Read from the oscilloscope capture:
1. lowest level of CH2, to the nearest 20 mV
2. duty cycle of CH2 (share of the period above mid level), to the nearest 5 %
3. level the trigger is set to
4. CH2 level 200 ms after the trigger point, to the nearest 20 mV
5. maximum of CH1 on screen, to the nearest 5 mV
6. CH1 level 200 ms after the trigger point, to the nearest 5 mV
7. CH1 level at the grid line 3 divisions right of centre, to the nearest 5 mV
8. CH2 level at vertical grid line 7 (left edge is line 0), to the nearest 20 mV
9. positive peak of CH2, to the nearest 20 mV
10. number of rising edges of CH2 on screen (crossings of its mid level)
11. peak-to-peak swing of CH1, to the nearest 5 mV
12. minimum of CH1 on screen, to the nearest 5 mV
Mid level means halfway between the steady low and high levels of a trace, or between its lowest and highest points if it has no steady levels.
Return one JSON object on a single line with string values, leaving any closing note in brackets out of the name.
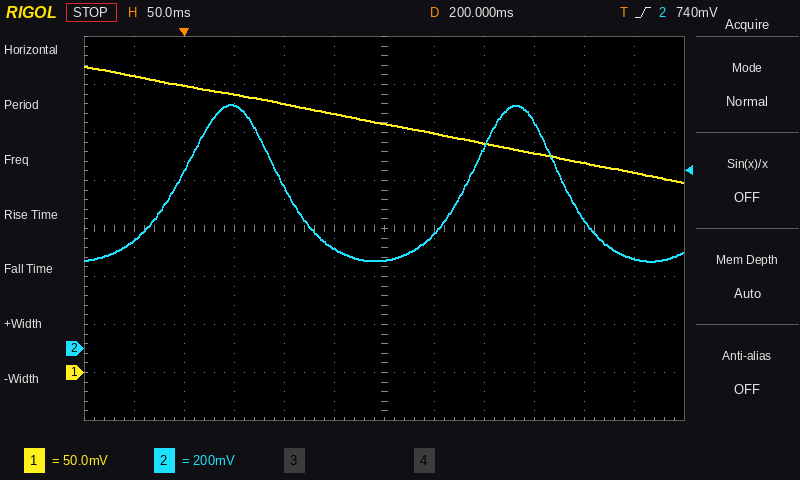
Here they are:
{"lowest level of CH2, to the nearest 20 mV": "360 mV", "duty cycle of CH2 (share of the period above mid level), to the nearest 5 %": "35 %", "level the trigger is set to": "740 mV", "CH2 level 200 ms after the trigger point, to the nearest 20 mV": "360 mV", "maximum of CH1 on screen, to the nearest 5 mV": "320 mV", "CH1 level 200 ms after the trigger point, to the nearest 5 mV": "260 mV", "CH1 level at the grid line 3 divisions right of centre, to the nearest 5 mV": "230 mV", "CH2 level at vertical grid line 7 (left edge is line 0), to the nearest 20 mV": "480 mV", "positive peak of CH2, to the nearest 20 mV": "1.02 V", "number of rising edges of CH2 on screen": "2", "peak-to-peak swing of CH1, to the nearest 5 mV": "120 mV", "minimum of CH1 on screen, to the nearest 5 mV": "200 mV"}
